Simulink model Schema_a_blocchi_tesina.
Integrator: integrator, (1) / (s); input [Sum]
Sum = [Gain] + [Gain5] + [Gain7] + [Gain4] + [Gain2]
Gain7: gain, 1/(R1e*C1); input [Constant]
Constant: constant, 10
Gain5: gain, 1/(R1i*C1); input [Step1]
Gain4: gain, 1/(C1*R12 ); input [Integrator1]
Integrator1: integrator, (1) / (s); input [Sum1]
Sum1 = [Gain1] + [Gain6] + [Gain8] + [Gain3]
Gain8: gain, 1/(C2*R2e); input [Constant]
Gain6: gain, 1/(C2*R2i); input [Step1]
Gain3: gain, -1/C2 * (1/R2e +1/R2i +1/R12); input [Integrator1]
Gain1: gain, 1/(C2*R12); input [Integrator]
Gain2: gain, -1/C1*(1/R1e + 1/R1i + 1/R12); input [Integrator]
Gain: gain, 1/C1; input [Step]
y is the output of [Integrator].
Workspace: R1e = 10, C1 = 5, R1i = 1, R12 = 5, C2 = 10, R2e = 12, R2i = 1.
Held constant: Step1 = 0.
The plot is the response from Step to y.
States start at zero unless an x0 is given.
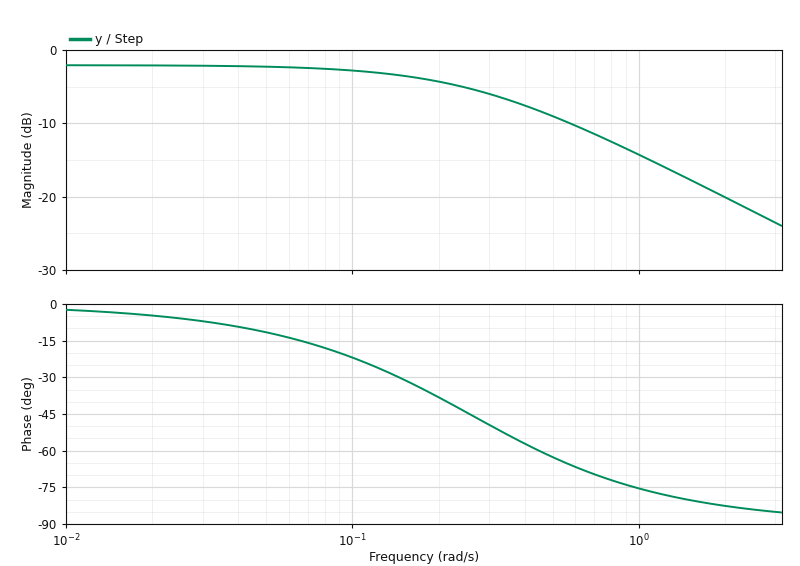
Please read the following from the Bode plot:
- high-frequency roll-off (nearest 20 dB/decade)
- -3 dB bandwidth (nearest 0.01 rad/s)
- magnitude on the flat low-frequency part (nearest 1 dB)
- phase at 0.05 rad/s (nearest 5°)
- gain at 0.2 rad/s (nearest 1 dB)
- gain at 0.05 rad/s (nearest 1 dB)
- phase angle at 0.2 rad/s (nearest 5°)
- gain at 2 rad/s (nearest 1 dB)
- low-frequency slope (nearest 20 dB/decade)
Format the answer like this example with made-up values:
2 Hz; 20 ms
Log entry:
-20 dB/decade; 0.25 rad/s; -2 dB; -10°; -4 dB; -2 dB; -40°; -20 dB; 0 dB/decade
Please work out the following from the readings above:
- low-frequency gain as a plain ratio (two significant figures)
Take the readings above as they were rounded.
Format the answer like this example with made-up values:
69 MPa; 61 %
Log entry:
0.79
